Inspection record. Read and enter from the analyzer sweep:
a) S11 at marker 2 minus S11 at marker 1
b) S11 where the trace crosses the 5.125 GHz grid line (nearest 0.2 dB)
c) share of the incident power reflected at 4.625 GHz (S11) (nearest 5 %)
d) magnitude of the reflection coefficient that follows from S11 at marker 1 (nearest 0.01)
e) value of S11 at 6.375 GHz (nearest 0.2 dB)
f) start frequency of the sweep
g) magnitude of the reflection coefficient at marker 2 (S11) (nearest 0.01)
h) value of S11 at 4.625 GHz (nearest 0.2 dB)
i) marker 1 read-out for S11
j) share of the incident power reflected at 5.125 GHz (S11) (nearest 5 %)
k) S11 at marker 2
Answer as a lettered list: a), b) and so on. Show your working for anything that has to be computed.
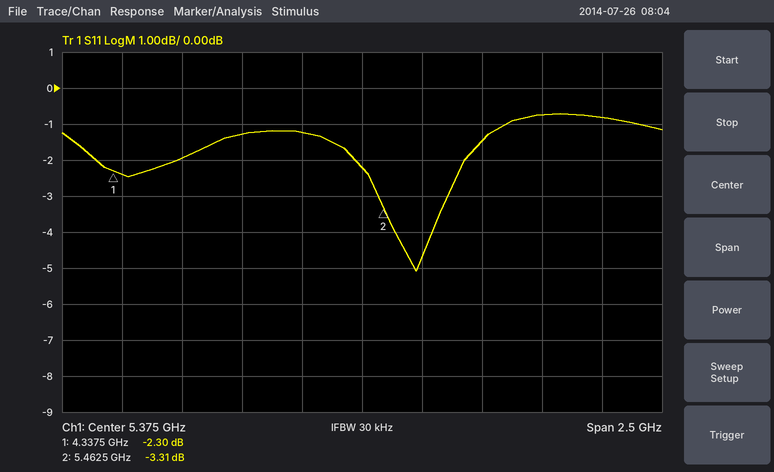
a) -3.31 − (-2.3) = -1.01 dB
b) -1.2 dB
c) 10^(-2/10) ≈ 63.1 %, so 65 % to the nearest 5 %
d) 10^(-2.3/20) ≈ 0.77
e) -0.8 dB
f) 4.125 GHz
g) 10^(-3.31/20) ≈ 0.68
h) -2.0 dB
i) -2.30 dB
j) 10^(-1.2/10) ≈ 75.9 %, so 75 % to the nearest 5 %
k) -3.31 dB
